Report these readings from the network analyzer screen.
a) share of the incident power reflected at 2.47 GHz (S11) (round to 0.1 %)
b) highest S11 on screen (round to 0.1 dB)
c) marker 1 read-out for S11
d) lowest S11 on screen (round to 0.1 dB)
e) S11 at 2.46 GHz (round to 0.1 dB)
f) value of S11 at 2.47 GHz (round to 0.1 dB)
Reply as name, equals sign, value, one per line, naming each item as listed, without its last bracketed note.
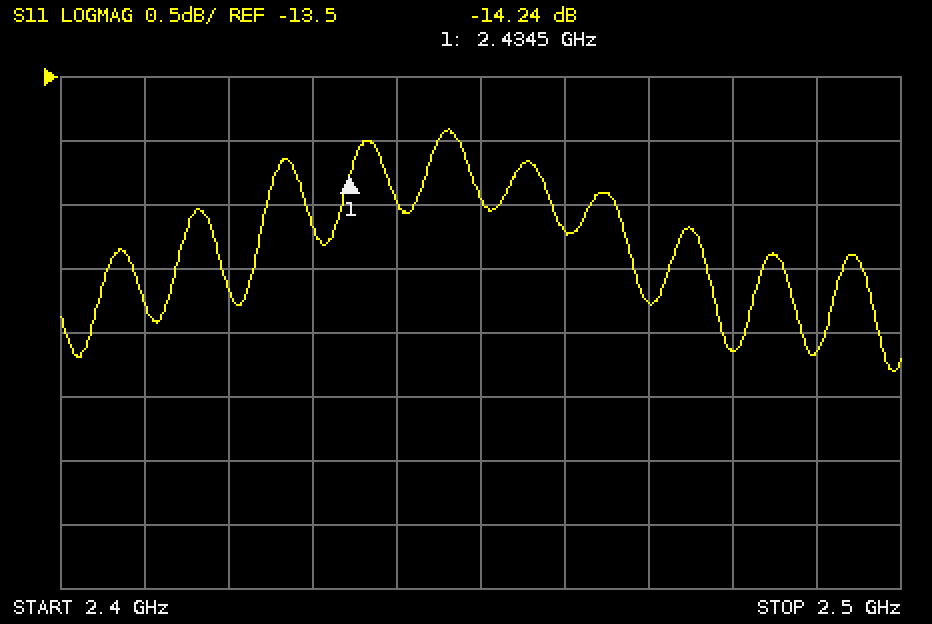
share of the incident power reflected at 2.47 GHz (S11) = 3.0 %
highest S11 on screen = -13.9 dB
marker 1 read-out for S11 = -14.24 dB
lowest S11 on screen = -15.8 dB
S11 at 2.46 GHz = -14.7 dB
value of S11 at 2.47 GHz = -15.3 dB
